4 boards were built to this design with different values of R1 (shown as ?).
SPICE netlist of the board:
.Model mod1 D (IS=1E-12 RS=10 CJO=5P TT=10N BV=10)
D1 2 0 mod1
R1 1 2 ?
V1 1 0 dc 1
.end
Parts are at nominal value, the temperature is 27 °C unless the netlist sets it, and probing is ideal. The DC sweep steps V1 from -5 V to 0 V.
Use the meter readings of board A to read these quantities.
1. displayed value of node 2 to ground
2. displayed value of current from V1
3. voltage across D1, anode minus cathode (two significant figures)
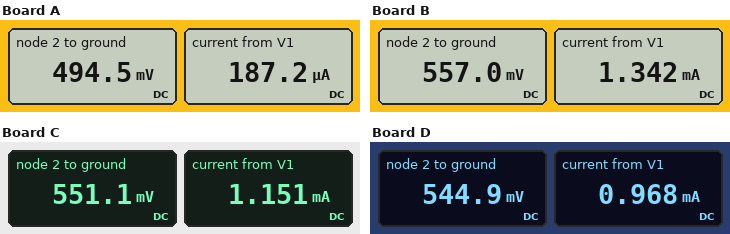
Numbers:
494.5 mV
187.2 µA
490 mV
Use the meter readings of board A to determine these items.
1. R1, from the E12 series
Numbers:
2.7 kΩ
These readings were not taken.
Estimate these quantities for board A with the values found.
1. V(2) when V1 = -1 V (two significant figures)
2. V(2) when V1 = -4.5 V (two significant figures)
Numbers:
-1.0 V
-4.5 V
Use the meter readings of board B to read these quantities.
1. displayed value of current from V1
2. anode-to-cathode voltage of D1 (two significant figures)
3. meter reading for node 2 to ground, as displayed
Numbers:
1.342 mA
560 mV
557.0 mV
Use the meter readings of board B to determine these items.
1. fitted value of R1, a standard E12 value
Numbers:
330 Ω
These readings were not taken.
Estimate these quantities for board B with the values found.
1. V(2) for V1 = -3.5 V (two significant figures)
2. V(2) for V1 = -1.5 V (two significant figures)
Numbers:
-3.5 V
-1.5 V
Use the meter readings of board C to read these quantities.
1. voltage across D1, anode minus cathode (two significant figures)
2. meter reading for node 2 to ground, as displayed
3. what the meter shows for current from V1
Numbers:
550 mV
551.1 mV
1.151 mA
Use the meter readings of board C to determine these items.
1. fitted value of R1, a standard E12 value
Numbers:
390 Ω
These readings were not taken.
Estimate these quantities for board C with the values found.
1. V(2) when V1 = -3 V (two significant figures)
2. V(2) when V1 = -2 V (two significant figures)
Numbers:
-3.0 V
-2.0 V
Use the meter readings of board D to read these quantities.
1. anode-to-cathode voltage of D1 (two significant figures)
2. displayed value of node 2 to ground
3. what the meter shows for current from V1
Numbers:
540 mV
544.9 mV
0.968 mA
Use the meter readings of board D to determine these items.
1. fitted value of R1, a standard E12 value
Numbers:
470 Ω
